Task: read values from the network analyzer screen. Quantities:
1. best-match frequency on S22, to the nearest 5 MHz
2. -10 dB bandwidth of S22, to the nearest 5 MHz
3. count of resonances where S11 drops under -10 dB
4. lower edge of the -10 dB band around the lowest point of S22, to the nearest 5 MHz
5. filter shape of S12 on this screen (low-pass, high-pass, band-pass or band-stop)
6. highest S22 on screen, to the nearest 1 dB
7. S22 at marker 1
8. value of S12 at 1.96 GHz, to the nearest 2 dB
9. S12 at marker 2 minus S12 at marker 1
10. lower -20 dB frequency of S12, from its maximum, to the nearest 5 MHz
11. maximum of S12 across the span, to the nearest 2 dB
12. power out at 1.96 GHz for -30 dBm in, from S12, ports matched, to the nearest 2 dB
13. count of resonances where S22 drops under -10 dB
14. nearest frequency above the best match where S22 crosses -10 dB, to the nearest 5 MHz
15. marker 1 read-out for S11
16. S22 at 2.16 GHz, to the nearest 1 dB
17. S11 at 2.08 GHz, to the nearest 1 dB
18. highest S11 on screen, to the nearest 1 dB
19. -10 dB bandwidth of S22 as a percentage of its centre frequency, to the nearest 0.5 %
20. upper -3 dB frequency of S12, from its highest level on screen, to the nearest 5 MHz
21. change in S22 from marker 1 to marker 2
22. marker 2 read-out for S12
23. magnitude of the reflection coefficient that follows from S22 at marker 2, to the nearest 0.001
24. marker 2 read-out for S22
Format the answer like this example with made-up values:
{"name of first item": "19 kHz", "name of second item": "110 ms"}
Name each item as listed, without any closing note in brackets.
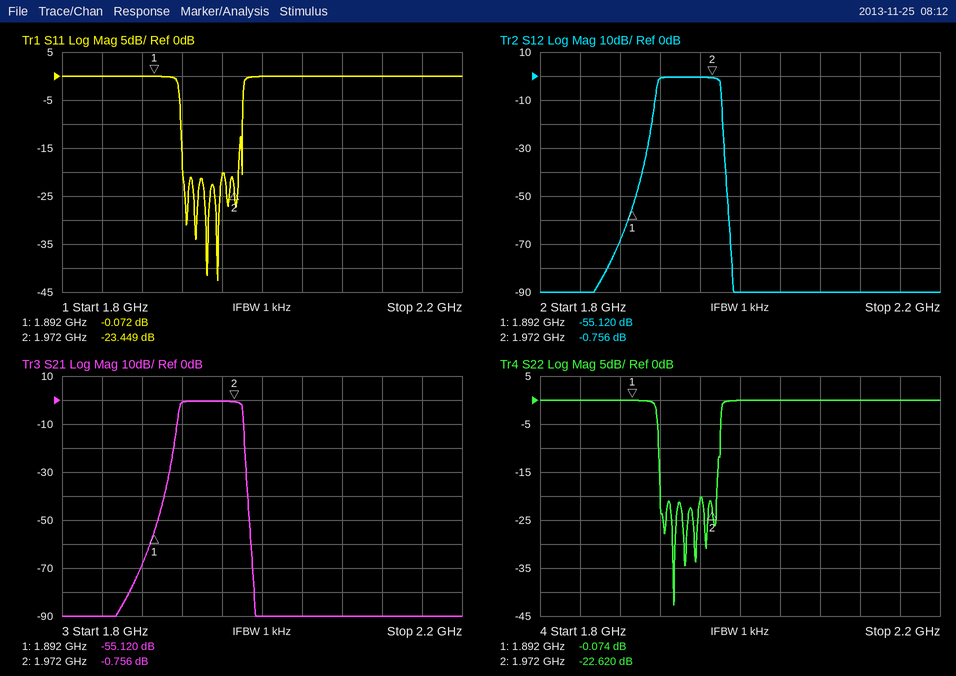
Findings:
{"best-match frequency on S22, to the nearest 5 MHz": "1.935 GHz", "-10 dB bandwidth of S22, to the nearest 5 MHz": "60 MHz", "count of resonances where S11 drops under -10 dB": "7", "lower edge of the -10 dB band around the lowest point of S22, to the nearest 5 MHz": "1.920 GHz", "filter shape of S12 on this screen": "band-pass", "highest S22 on screen, to the nearest 1 dB": "0 dB", "S22 at marker 1": "-0.074 dB", "value of S12 at 1.96 GHz, to the nearest 2 dB": "0 dB", "S12 at marker 2 minus S12 at marker 1": "54.364 dB", "lower -20 dB frequency of S12, from its maximum, to the nearest 5 MHz": "1.910 GHz", "maximum of S12 across the span, to the nearest 2 dB": "0 dB", "power out at 1.96 GHz for -30 dBm in, from S12, ports matched, to the nearest 2 dB": "-30 dBm", "count of resonances where S22 drops under -10 dB": "6", "nearest frequency above the best match where S22 crosses -10 dB, to the nearest 5 MHz": "1.980 GHz", "marker 1 read-out for S11": "-0.072 dB", "S22 at 2.16 GHz, to the nearest 1 dB": "0 dB", "S11 at 2.08 GHz, to the nearest 1 dB": "0 dB", "highest S11 on screen, to the nearest 1 dB": "0 dB", "-10 dB bandwidth of S22 as a percentage of its centre frequency, to the nearest 0.5 %": "3.0 %", "upper -3 dB frequency of S12, from its highest level on screen, to the nearest 5 MHz": "1.980 GHz", "change in S22 from marker 1 to marker 2": "-22.546 dB", "marker 2 read-out for S12": "-0.756 dB", "magnitude of the reflection coefficient that follows from S22 at marker 2, to the nearest 0.001": "0.074", "marker 2 read-out for S22": "-22.620 dB"}
